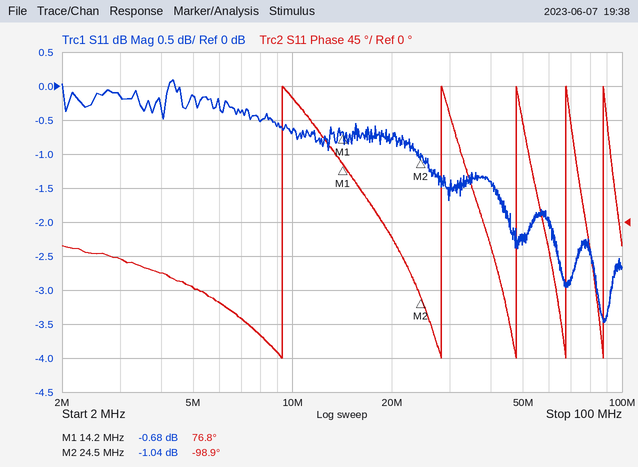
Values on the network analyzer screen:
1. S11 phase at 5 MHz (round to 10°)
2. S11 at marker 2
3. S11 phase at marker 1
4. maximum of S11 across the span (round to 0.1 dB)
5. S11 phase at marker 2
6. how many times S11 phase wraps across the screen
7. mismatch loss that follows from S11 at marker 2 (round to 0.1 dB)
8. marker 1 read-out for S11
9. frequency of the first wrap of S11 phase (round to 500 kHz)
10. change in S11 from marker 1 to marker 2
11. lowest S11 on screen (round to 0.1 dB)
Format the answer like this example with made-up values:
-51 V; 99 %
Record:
-90°; -1.04 dB; 76.8°; 0.1 dB; -98.9°; 5; 6.7 dB; -0.68 dB; 9.5 MHz; -0.36 dB; -3.5 dB
